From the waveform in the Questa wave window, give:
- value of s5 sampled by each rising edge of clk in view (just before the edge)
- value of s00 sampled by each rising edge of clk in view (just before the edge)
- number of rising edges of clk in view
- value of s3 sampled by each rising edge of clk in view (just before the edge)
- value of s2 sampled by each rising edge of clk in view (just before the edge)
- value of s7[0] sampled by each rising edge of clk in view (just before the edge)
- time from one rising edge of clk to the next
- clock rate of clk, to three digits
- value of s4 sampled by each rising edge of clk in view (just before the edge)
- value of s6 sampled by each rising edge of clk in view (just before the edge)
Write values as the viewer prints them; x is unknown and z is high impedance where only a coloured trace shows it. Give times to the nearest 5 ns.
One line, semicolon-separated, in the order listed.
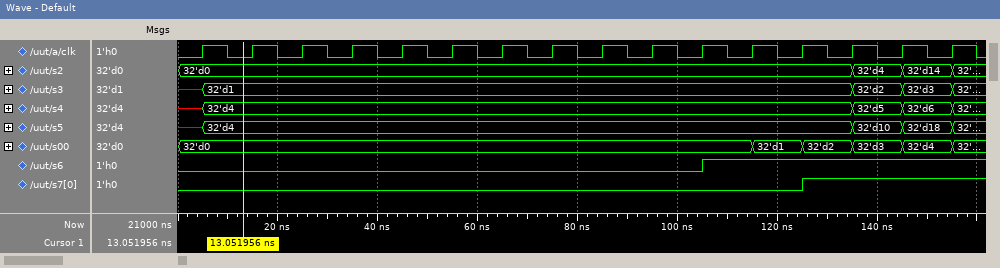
x, 32'd4, 32'd4, 32'd4, 32'd4, 32'd4, 32'd4, 32'd4, 32'd4, 32'd4, 32'd4, 32'd4, 32'd4, 32'd4, 32'd10, 32'd18; 32'd0, 32'd0, 32'd0, 32'd0, 32'd0, 32'd0, 32'd0, 32'd0, 32'd0, 32'd0, 32'd0, 32'd0, 32'd1, 32'd2, 32'd3, 32'd4; 16; x, 32'd1, 32'd1, 32'd1, 32'd1, 32'd1, 32'd1, 32'd1, 32'd1, 32'd1, 32'd1, 32'd1, 32'd1, 32'd1, 32'd2, 32'd3; 32'd0, 32'd0, 32'd0, 32'd0, 32'd0, 32'd0, 32'd0, 32'd0, 32'd0, 32'd0, 32'd0, 32'd0, 32'd0, 32'd0, 32'd4, 32'd14; 0 0 0 0 0 0 0 0 0 0 0 0 0 1 1 1; 10 ns; 100 MHz; x, 32'd4, 32'd4, 32'd4, 32'd4, 32'd4, 32'd4, 32'd4, 32'd4, 32'd4, 32'd4, 32'd4, 32'd4, 32'd4, 32'd5, 32'd6; 0 0 0 0 0 0 0 0 0 0 0 1 1 1 1 1
